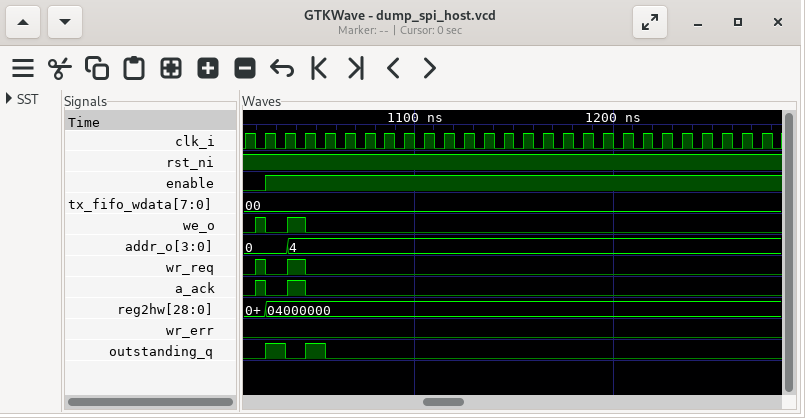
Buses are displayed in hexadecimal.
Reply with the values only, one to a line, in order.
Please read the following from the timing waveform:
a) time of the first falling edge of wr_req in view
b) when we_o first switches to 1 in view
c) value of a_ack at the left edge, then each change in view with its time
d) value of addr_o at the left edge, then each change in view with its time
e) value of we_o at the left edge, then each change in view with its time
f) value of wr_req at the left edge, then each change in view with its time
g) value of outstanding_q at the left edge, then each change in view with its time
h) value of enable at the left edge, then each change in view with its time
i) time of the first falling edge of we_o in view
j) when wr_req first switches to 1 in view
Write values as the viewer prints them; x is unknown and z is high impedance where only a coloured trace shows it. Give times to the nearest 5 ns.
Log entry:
1025 ns
1020 ns
0, 1 at 1020 ns, 0 at 1025 ns, 1 at 1035 ns, 0 at 1045 ns
0, 4 at 1035 ns
0, 1 at 1020 ns, 0 at 1025 ns, 1 at 1035 ns, 0 at 1045 ns
0, 1 at 1020 ns, 0 at 1025 ns, 1 at 1035 ns, 0 at 1045 ns
0, 1 at 1025 ns, 0 at 1035 ns, 1 at 1045 ns, 0 at 1055 ns
0, 1 at 1025 ns
1025 ns
1020 ns
